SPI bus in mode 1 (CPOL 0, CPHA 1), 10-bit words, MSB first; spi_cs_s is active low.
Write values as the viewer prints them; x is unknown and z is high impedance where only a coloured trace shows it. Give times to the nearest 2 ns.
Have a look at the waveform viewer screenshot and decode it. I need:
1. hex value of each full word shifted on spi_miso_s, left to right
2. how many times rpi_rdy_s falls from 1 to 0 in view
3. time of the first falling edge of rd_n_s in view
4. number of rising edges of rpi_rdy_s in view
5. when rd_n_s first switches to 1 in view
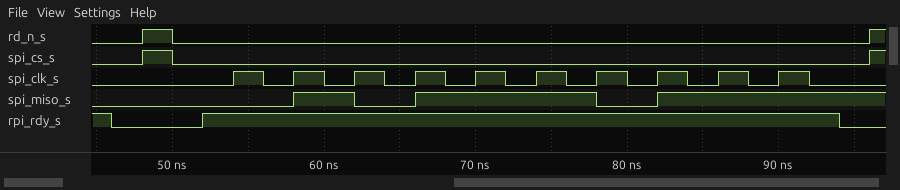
177
2
50 ns
1
48 ns
